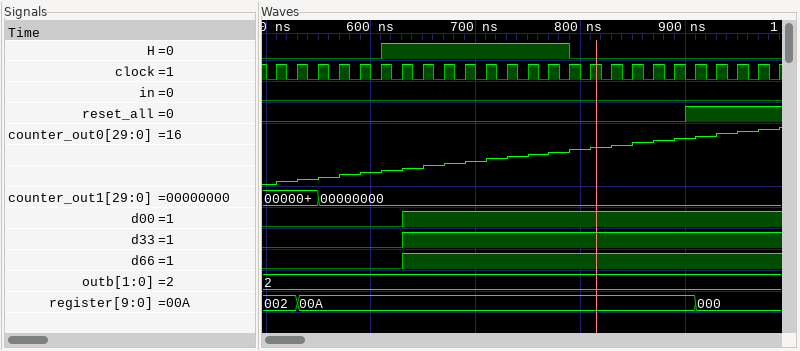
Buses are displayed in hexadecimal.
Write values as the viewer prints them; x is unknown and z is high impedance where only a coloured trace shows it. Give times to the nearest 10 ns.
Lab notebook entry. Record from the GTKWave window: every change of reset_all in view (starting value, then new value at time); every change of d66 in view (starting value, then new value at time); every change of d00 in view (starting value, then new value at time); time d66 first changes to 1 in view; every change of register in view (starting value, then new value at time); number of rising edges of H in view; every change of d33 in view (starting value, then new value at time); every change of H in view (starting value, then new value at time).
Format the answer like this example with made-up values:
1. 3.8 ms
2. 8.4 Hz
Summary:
1. 0, 1 at 900 ns
2. 0, 1 at 630 ns
3. 0, 1 at 630 ns
4. 630 ns
5. 002, 00A at 530 ns, 000 at 910 ns
6. 1
7. 0, 1 at 630 ns
8. 0, 1 at 610 ns, 0 at 790 ns
